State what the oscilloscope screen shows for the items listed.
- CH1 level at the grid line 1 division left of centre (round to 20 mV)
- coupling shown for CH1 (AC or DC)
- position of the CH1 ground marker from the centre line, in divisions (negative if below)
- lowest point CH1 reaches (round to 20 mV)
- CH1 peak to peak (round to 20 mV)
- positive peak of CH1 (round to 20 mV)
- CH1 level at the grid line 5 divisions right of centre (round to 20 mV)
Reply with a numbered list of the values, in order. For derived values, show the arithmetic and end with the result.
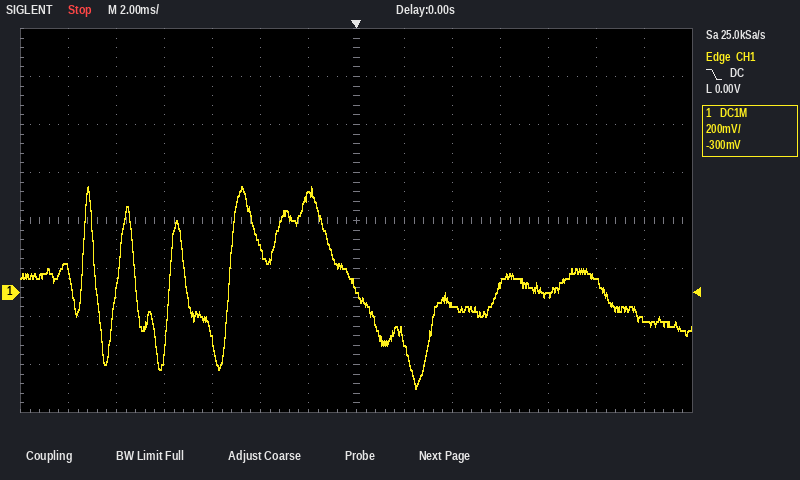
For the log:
1. 400 mV
2. DC
3. -1.5 div
4. -400 mV
5. 440 mV − (-400 mV) = 840 mV
6. 440 mV
7. 60 mV
